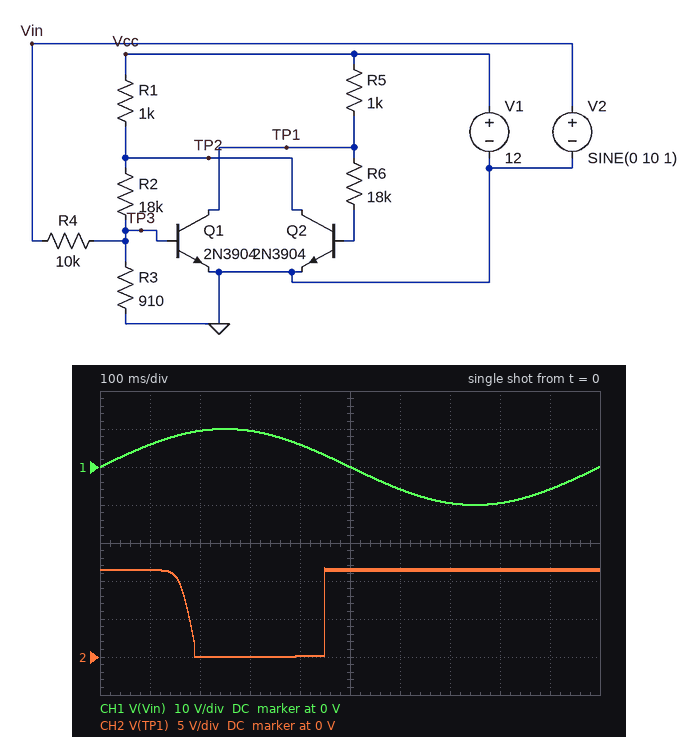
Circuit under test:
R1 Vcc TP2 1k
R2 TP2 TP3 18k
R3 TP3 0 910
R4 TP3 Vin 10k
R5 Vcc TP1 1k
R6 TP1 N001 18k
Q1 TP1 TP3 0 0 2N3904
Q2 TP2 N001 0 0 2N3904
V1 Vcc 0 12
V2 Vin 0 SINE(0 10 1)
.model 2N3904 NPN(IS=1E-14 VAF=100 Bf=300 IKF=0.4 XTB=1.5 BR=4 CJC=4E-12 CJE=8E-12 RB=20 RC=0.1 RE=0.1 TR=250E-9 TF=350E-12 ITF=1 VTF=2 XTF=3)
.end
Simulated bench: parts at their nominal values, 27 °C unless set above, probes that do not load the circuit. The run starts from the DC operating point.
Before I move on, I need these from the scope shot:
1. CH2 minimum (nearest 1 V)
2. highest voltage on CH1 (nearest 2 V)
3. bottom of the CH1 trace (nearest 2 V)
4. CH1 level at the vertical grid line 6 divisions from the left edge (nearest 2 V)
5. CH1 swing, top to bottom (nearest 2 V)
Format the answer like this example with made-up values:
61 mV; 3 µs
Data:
0 V; 10 V; -10 V; -6 V; 20 V
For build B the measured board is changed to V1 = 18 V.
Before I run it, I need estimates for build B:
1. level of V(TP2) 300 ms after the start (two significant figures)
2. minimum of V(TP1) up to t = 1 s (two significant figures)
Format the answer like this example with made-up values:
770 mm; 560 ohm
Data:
17 V; 52 mV
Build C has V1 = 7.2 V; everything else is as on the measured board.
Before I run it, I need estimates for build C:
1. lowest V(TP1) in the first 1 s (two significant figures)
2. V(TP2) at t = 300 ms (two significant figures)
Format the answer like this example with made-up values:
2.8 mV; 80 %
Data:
45 mV; 6.9 V
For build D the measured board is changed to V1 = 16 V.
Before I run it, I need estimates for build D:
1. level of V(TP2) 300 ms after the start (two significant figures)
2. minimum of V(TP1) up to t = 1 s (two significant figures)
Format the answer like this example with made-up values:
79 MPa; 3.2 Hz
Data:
15 V; 51 mV
